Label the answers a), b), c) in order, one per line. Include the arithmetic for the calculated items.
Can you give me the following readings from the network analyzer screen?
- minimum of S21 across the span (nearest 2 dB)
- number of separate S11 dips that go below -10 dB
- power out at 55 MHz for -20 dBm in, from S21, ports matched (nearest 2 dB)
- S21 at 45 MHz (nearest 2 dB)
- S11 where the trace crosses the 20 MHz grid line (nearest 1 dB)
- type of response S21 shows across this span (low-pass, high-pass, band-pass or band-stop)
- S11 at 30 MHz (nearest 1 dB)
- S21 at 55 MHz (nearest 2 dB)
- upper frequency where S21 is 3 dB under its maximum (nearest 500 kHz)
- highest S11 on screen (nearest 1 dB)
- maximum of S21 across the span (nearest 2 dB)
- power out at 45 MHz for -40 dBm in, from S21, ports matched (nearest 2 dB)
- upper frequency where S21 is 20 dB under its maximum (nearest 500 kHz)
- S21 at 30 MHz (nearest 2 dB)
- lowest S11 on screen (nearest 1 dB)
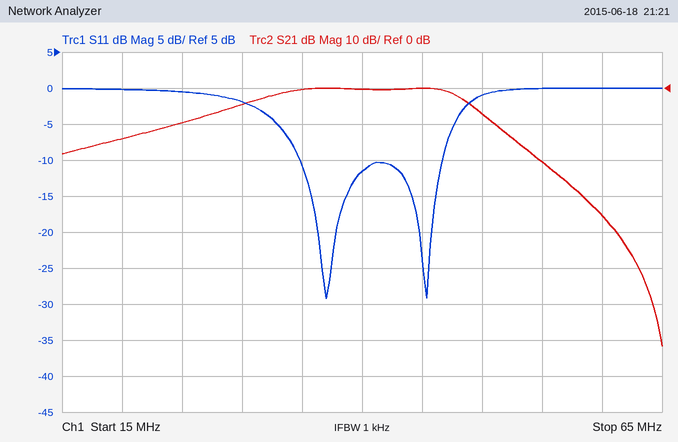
a) -72 dB
b) 2
c) -20 dBm + (-20 dB) = -40 dBm
d) 0 dB
e) 0 dB
f) band-pass
g) -2 dB
h) -20 dB
i) 48.5 MHz
j) 0 dB
k) 0 dB
l) -40 dBm + (0 dB) = -40 dBm
m) 55.0 MHz
n) -4 dB
o) -29 dB
